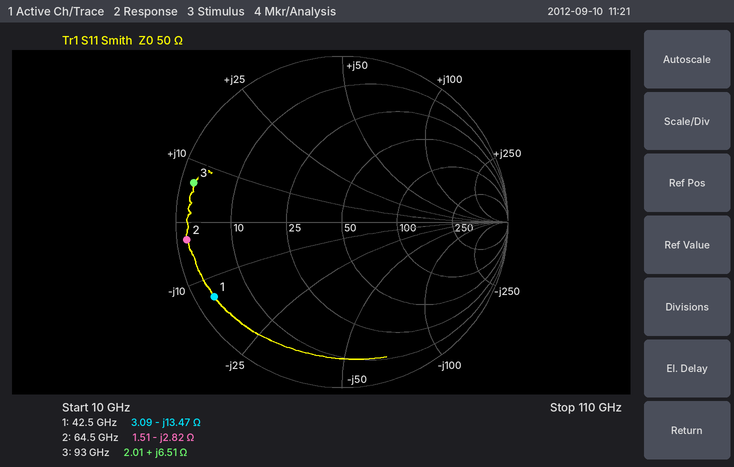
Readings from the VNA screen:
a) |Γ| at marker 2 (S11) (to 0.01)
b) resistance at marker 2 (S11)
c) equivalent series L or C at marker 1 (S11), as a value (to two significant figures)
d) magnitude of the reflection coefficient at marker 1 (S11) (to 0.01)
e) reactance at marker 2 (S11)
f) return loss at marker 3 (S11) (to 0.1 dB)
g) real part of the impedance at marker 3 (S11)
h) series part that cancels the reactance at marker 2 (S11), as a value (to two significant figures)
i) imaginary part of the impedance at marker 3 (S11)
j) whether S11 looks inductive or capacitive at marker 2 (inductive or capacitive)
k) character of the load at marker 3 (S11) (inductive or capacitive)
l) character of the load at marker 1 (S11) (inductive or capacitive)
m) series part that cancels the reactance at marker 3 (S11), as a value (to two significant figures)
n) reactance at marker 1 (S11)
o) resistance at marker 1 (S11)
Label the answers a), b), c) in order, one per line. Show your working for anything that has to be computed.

a) 0.94
b) 1.51 Ω
c) C = 1/(2π × 42.5 GHz × 13.47 Ω) ≈ 278 fF, so 280 fF to two significant figures
d) 0.89
e) -2.82 Ω
f) 0.7 dB
g) 2.01 Ω
h) L = 2.82 Ω/(2π × 64.5 GHz) ≈ 7.0 pH
i) +6.51 Ω
j) capacitive
k) inductive
l) capacitive
m) C = 1/(2π × 93 GHz × 6.51 Ω) ≈ 263 fF, so 260 fF to two significant figures
n) -13.47 Ω
o) 3.09 Ω
